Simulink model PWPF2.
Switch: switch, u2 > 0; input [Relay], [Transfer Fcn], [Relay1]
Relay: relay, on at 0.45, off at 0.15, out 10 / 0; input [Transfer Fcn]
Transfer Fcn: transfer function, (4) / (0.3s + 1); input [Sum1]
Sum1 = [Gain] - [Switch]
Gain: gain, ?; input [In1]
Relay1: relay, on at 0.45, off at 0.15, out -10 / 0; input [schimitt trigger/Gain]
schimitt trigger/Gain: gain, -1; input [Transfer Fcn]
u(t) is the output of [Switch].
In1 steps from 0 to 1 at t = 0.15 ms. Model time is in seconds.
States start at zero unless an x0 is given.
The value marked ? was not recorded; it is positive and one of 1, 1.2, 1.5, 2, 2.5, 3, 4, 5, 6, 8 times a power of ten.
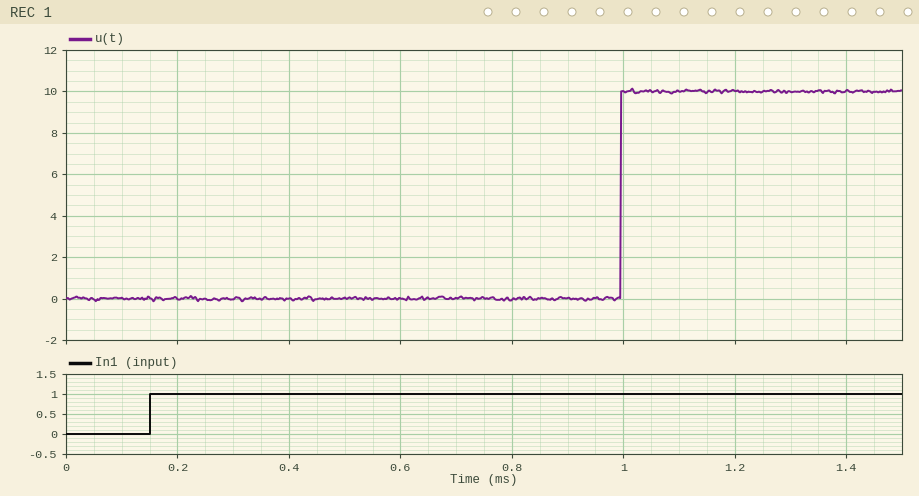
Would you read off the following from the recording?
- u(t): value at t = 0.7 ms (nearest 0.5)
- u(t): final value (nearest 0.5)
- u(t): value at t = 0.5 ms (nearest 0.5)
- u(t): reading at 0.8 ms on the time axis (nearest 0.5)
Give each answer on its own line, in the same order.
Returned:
0.0
10.0
0.0
0.0
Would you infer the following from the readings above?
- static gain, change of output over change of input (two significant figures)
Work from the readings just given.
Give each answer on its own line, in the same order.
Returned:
10
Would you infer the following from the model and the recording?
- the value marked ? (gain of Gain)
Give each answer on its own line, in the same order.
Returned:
40
